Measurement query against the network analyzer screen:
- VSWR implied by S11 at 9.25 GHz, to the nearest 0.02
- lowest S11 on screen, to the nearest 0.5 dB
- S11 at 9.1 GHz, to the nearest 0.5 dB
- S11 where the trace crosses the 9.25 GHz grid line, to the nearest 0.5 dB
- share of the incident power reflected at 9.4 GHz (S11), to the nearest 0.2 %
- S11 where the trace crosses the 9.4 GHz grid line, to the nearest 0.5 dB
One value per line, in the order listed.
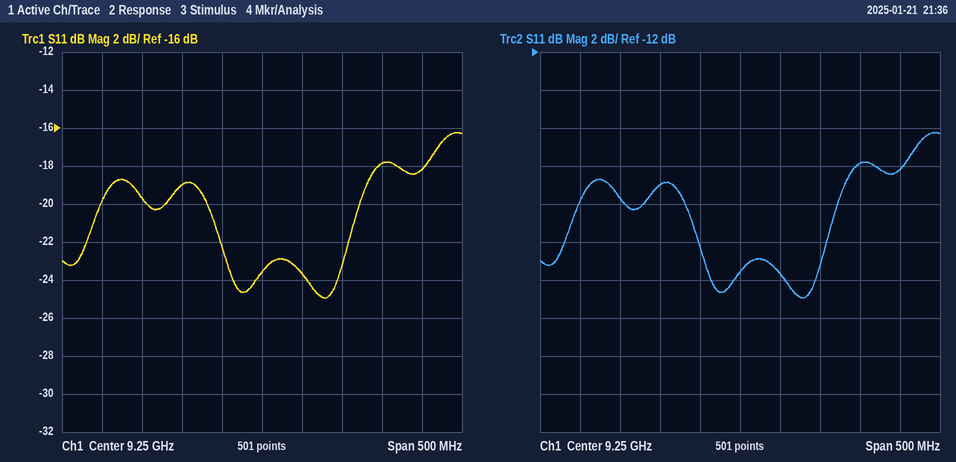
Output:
1.14
-25.0 dB
-19.5 dB
-23.5 dB
1.6 %
-18.0 dB
